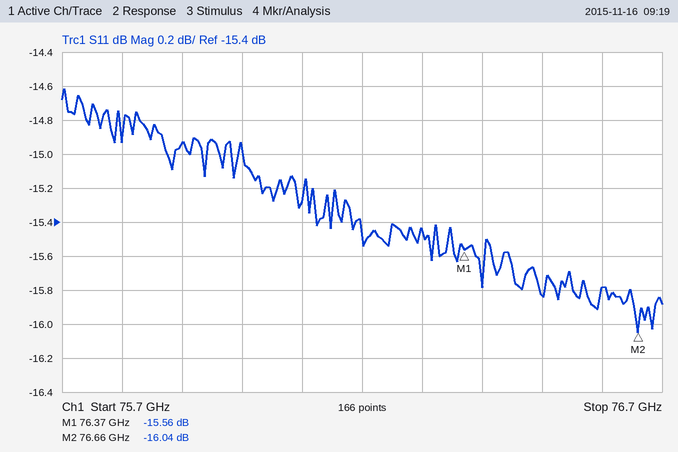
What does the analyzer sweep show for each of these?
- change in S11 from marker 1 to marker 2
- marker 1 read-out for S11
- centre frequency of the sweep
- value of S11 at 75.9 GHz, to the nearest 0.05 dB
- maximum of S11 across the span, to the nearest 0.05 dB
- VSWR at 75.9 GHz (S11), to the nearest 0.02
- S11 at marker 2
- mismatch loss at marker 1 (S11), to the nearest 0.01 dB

-0.48 dB
-15.56 dB
76.2 GHz
-14.95 dB
-14.60 dB
1.44
-16.04 dB
0.12 dB
